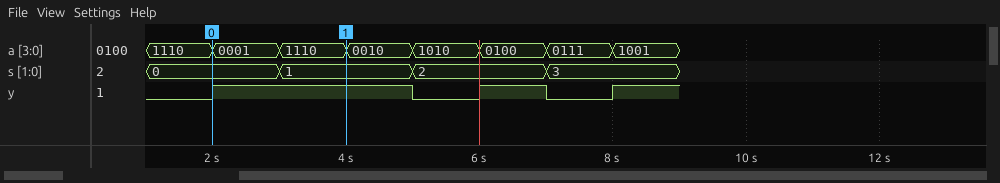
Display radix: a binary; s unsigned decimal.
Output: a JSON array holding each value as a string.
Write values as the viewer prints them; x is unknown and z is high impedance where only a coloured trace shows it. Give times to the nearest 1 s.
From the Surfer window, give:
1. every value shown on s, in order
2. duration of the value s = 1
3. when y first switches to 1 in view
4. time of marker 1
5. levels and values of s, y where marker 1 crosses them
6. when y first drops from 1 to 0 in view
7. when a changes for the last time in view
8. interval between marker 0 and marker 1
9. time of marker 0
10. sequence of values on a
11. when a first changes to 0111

["0, 1, 2, 3", "2 s", "2 s", "4 s", "s=1, y=1", "5 s", "8 s", "2 s", "2 s", "1110, 0001, 1110, 0010, 1010, 0100, 0111, 1001", "7 s"]
